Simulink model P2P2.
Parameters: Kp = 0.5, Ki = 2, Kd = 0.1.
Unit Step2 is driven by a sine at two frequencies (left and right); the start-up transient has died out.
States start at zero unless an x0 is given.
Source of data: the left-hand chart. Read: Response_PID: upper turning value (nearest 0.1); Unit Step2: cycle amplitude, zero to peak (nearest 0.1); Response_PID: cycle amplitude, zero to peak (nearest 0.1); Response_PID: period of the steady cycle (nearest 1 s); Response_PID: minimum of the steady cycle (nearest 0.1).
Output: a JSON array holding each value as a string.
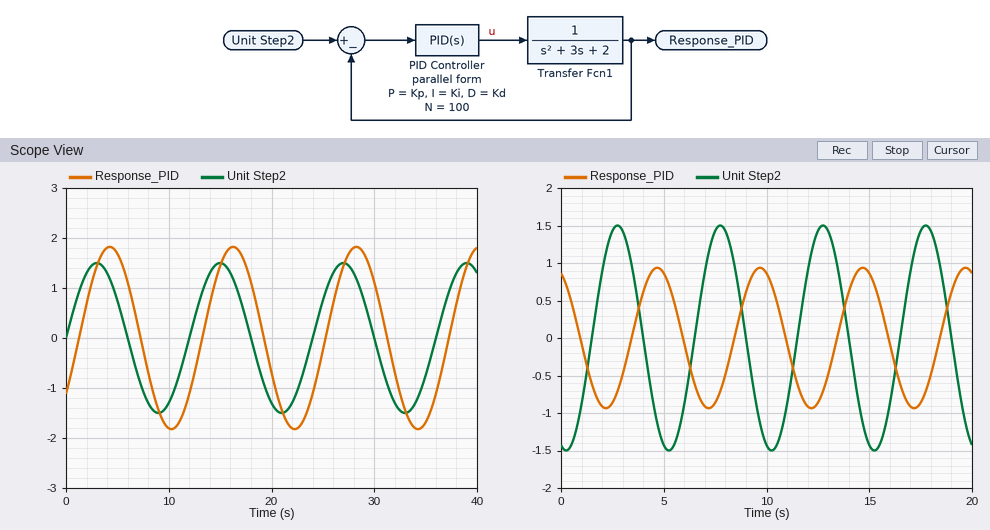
["1.8", "1.5", "1.8", "12 s", "-1.8"]
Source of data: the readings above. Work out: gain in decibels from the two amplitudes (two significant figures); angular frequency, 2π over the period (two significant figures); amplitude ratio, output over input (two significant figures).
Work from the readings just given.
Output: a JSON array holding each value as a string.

["1.6 dB", "0.52 rad/s", "1.2"]
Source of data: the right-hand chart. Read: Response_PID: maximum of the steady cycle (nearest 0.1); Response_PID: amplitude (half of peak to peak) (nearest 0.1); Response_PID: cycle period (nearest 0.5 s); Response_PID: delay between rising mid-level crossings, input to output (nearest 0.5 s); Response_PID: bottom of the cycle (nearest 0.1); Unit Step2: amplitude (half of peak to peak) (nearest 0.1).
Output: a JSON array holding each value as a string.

["0.9", "0.9", "5.0 s", "2.0 s", "-0.9", "1.5"]
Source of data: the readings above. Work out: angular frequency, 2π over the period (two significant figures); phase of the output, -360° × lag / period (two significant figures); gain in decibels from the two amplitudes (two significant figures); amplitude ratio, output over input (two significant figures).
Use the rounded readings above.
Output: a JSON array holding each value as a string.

["1.3 rad/s", "-140°", "-4.4 dB", "0.60"]
